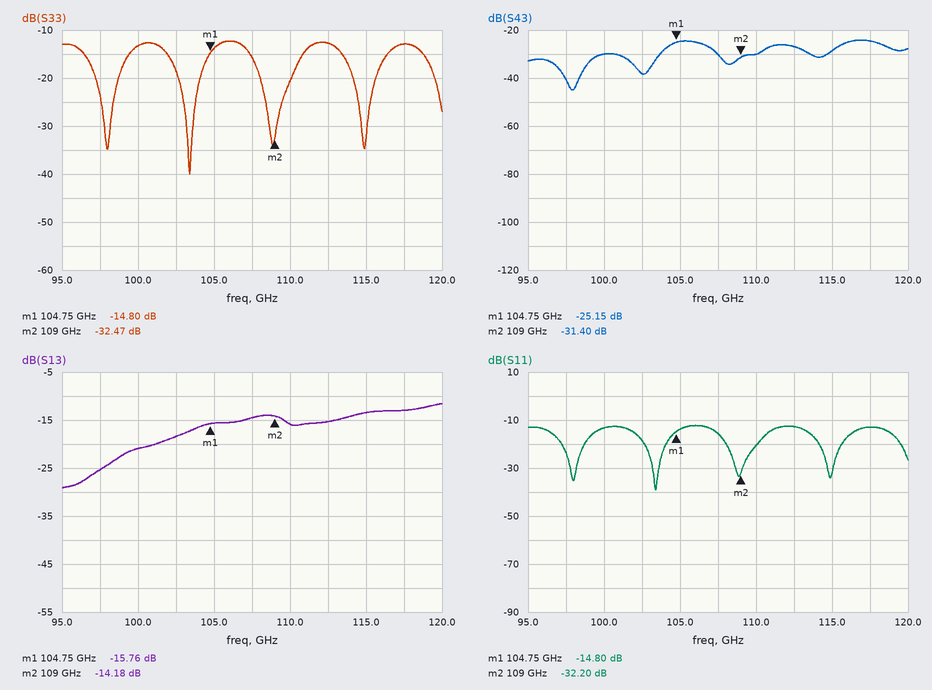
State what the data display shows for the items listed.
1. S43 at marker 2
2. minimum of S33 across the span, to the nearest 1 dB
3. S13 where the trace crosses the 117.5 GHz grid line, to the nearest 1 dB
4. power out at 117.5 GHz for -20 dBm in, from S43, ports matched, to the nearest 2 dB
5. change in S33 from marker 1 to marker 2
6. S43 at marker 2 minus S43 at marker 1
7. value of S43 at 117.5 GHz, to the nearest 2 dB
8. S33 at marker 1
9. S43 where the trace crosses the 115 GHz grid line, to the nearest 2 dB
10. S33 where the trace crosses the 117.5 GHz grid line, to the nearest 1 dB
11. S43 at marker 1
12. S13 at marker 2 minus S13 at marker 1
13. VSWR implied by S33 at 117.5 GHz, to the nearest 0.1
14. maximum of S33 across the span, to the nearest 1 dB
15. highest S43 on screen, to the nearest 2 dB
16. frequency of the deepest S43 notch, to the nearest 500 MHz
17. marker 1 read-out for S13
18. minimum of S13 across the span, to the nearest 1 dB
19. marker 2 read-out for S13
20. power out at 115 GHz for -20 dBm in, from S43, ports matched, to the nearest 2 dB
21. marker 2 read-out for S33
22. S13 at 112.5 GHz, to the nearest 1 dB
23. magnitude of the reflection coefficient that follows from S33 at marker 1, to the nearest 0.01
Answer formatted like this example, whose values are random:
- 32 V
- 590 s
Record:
- -31.40 dB
- -40 dB
- -13 dB
- -44 dBm
- -17.67 dB
- -6.25 dB
- -24 dB
- -14.80 dB
- -28 dB
- -13 dB
- -25.15 dB
- 1.58 dB
- 1.6
- -12 dB
- -24 dB
- 98.0 GHz
- -15.76 dB
- -29 dB
- -14.18 dB
- -48 dBm
- -32.47 dB
- -15 dB
- 0.18
